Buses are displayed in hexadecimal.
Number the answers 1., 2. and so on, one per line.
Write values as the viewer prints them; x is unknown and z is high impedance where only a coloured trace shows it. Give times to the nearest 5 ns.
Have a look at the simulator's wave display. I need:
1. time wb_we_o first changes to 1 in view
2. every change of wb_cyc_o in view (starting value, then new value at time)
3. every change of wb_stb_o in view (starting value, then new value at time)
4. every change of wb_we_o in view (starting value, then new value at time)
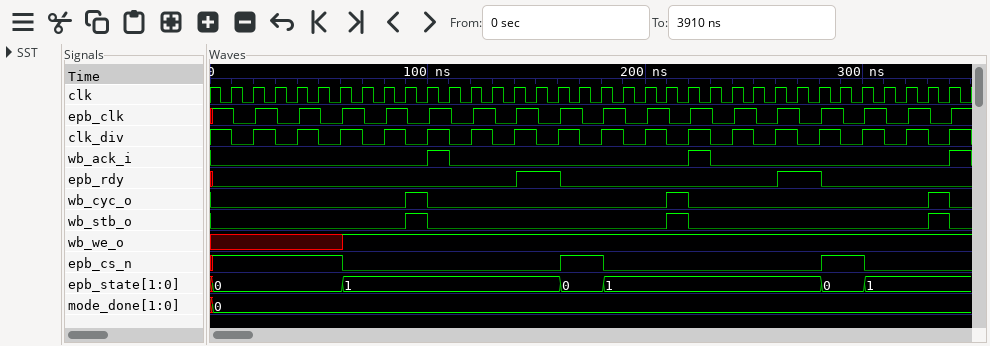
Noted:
1. 60 ns
2. 0, 1 at 90 ns, 0 at 100 ns, 1 at 210 ns, 0 at 220 ns, 1 at 330 ns, 0 at 340 ns
3. 0, 1 at 90 ns, 0 at 100 ns, 1 at 210 ns, 0 at 220 ns, 1 at 330 ns, 0 at 340 ns
4. x, 1 at 60 ns
